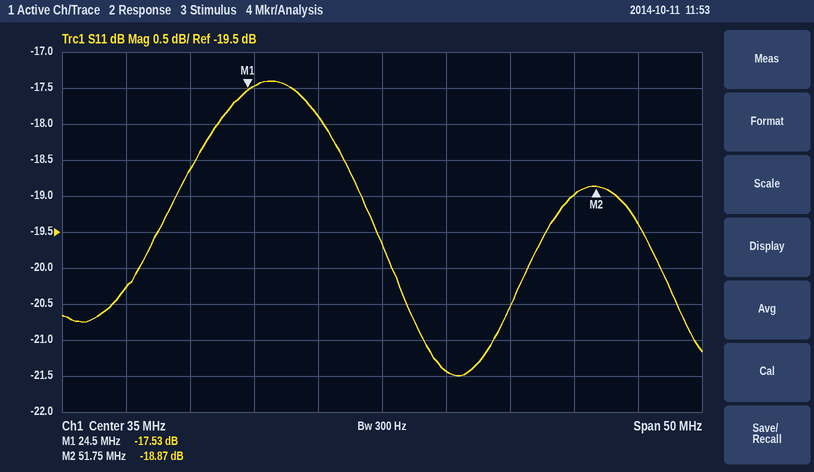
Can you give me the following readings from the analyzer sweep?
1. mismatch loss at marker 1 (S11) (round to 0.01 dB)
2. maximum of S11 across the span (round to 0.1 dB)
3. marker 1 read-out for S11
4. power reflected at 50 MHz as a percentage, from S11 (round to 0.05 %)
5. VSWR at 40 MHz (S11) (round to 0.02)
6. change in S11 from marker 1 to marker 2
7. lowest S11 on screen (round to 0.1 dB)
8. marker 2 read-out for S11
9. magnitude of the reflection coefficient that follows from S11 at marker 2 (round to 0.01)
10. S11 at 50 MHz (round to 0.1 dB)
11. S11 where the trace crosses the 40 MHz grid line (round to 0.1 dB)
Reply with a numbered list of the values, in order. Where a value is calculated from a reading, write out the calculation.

1. −10 log10(1 − 10^(-17.53/10)) ≈ 0.08 dB
2. -17.4 dB
3. -17.53 dB
4. 10^(-19/10) ≈ 1.26 %, so 1.25 % to the nearest 0.05 %
5. |Γ| = 10^(-21.4/20) = 0.0851; VSWR = (1 + 0.0851)/(1 − 0.0851) ≈ 1.19, so 1.18 to the nearest 0.02
6. -18.87 − (-17.53) = -1.34 dB
7. -21.5 dB
8. -18.87 dB
9. 10^(-18.87/20) ≈ 0.11
10. -19.0 dB
11. -21.4 dB
